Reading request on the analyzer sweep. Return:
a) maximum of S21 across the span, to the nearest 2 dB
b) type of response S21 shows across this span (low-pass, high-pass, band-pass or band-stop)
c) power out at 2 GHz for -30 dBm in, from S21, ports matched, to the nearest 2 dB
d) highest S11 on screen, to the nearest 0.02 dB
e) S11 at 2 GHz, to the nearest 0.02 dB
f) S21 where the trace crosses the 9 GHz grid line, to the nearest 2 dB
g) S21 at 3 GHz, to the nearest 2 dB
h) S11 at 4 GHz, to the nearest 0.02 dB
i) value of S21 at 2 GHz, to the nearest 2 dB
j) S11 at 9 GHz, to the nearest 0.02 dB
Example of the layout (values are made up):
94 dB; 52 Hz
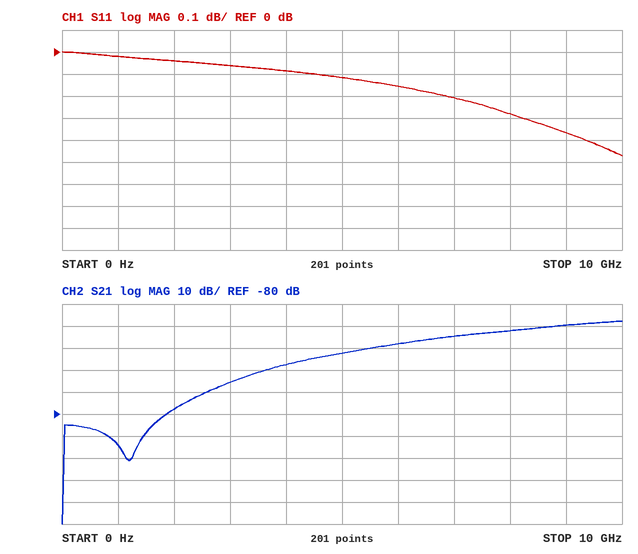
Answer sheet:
-38 dB; high-pass; -108 dBm; 0.00 dB; -0.04 dB; -40 dB; -66 dB; -0.08 dB; -78 dB; -0.36 dB
